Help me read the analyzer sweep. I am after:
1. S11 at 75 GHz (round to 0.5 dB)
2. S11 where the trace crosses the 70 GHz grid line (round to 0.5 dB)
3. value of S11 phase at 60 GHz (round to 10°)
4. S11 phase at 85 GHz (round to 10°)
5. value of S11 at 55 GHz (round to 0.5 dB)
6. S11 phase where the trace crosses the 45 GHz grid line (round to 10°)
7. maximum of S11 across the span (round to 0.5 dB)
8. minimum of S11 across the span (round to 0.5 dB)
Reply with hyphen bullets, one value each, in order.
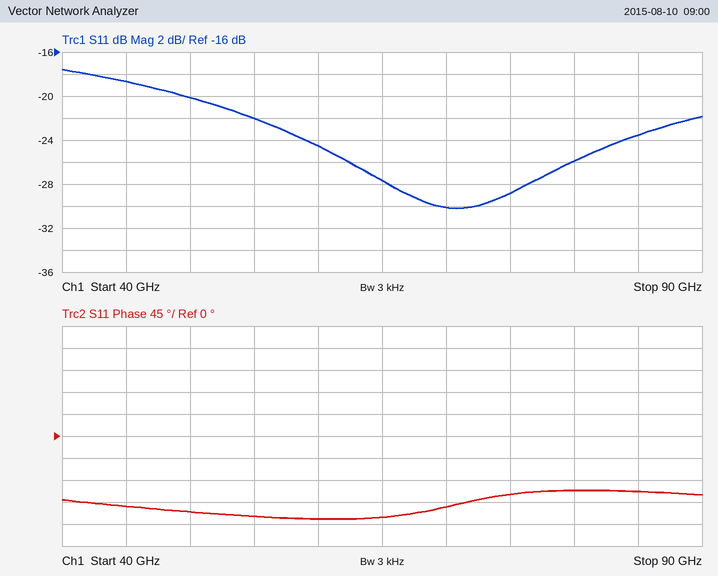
- -29.0 dB
- -30.0 dB
- -170°
- -110°
- -22.0 dB
- -140°
- -17.5 dB
- -30.0 dB
